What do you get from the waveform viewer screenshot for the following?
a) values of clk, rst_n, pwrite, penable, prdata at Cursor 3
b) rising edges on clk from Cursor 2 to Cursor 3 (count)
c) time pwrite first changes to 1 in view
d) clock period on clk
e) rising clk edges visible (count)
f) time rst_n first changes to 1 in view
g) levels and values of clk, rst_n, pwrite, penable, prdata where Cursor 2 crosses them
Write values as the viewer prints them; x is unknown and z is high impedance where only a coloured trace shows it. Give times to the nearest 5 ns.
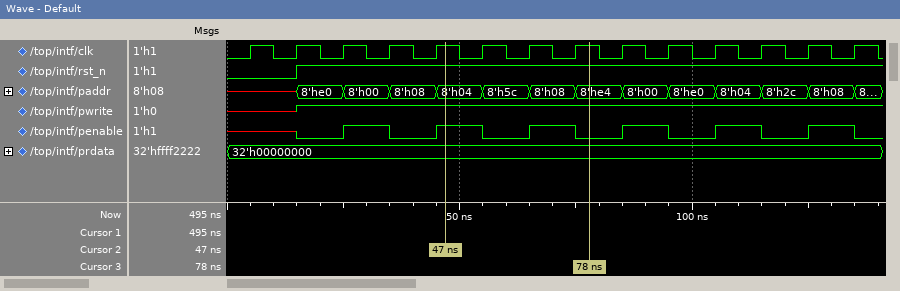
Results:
clk=1, rst_n=1, pwrite=1, penable=0, prdata=32'h00000000
3
15 ns
10 ns
14
15 ns
clk=1, rst_n=1, pwrite=1, penable=1, prdata=32'h00000000
